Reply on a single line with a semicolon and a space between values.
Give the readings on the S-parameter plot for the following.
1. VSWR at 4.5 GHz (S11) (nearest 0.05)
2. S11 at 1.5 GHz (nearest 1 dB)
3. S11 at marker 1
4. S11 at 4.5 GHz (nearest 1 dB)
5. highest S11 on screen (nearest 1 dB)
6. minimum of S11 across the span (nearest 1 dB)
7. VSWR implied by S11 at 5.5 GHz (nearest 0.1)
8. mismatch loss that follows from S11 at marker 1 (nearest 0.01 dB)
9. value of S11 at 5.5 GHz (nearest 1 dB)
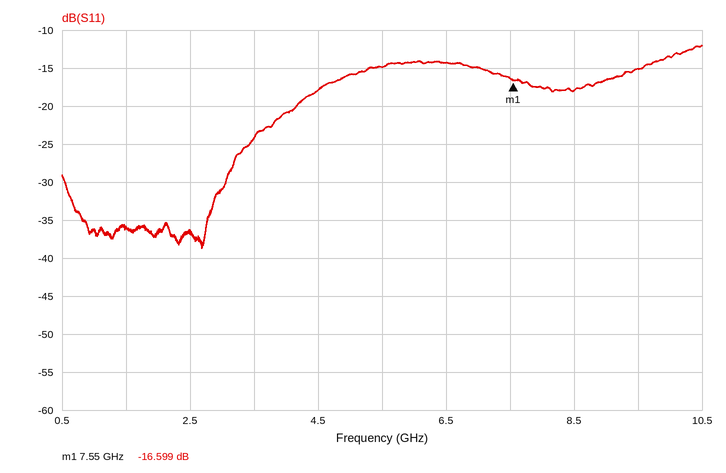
1.30; -36 dB; -16.599 dB; -18 dB; -12 dB; -39 dB; 1.4; 0.10 dB; -15 dB
